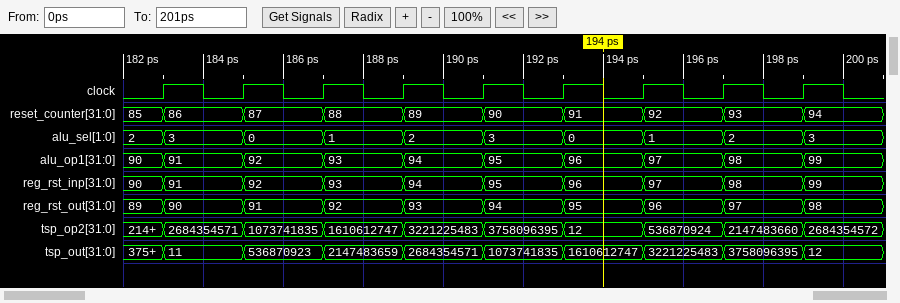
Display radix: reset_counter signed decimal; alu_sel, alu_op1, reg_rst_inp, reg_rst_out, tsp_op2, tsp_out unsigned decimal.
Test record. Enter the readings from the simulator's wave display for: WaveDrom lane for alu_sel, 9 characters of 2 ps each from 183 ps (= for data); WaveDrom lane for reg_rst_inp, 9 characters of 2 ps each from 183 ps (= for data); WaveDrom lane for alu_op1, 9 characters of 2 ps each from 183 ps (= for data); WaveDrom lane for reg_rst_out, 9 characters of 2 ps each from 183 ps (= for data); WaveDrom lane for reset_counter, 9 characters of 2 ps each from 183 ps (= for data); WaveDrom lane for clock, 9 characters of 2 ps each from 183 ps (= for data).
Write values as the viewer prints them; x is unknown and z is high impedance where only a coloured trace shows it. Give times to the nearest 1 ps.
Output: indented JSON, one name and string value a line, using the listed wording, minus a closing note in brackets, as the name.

{
  "WaveDrom lane for alu_sel, 9 characters of 2 ps each from 183 ps": "{name: 'alu_sel', wave: '=========', data: '3 0 1 2 3 0 1 2 3'}",
  "WaveDrom lane for reg_rst_inp, 9 characters of 2 ps each from 183 ps": "{name: 'reg_rst_inp', wave: '=========', data: '91 92 93 94 95 96 97 98 99'}",
  "WaveDrom lane for alu_op1, 9 characters of 2 ps each from 183 ps": "{name: 'alu_op1', wave: '=========', data: '91 92 93 94 95 96 97 98 99'}",
  "WaveDrom lane for reg_rst_out, 9 characters of 2 ps each from 183 ps": "{name: 'reg_rst_out', wave: '=========', data: '90 91 92 93 94 95 96 97 98'}",
  "WaveDrom lane for reset_counter, 9 characters of 2 ps each from 183 ps": "{name: 'reset_counter', wave: '=========', data: '86 87 88 89 90 91 92 93 94'}",
  "WaveDrom lane for clock, 9 characters of 2 ps each from 183 ps": "{name: 'clock', wave: 'p........'}"
}
